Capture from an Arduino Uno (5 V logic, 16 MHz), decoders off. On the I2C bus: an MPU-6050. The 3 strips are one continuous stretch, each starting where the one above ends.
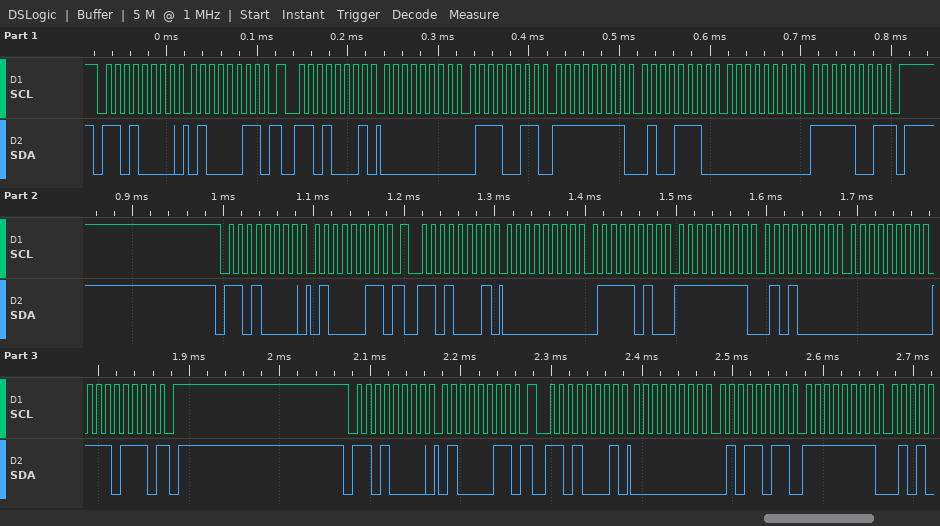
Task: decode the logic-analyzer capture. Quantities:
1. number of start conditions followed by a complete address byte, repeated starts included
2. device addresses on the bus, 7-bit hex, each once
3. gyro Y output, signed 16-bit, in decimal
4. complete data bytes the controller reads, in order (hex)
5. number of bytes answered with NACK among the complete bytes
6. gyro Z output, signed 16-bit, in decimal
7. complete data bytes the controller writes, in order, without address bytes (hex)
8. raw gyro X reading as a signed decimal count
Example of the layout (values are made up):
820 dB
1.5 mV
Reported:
6
0x68
-178
00 73 FF 4E 00 F9 00 7A FF 50 00 EE 00 5B FF
2
249
43 43 43
115
